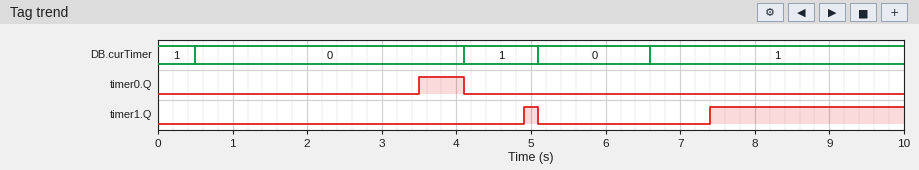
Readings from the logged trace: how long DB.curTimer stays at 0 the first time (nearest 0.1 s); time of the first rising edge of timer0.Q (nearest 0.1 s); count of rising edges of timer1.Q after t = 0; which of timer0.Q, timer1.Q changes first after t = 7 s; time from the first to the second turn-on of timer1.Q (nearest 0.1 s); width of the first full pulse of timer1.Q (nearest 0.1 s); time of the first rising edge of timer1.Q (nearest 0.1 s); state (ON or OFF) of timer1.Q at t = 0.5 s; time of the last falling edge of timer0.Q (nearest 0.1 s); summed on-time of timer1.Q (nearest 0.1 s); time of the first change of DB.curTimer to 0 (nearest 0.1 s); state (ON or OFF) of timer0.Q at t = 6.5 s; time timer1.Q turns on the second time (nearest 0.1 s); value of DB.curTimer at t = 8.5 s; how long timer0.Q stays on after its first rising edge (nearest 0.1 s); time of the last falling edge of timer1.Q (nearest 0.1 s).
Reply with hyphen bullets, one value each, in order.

- 3.6 s
- 3.5 s
- 2
- timer1.Q
- 2.5 s
- 0.2 s
- 4.9 s
- OFF
- 4.1 s
- 2.8 s
- 0.5 s
- OFF
- 7.4 s
- 1
- 0.6 s
- 5.1 s
